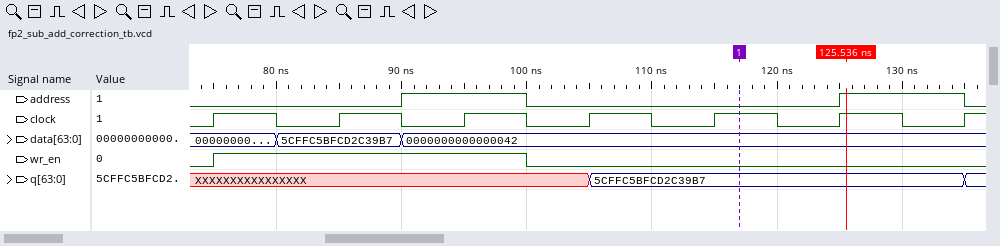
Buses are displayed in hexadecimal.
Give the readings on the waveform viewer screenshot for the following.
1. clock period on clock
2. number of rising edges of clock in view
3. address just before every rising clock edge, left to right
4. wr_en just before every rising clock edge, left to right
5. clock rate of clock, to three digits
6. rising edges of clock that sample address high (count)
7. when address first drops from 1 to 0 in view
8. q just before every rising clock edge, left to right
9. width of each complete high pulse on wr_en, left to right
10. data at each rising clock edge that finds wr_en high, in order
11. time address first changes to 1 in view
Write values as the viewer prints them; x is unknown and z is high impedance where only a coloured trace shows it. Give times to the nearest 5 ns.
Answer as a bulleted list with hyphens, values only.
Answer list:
- 10 ns
- 7
- 0 0 1 0 0 0 1
- 0 1 1 0 0 0 0
- 100 MHz
- 2
- 100 ns
- XXXXXXXXXXXXXXXX, XXXXXXXXXXXXXXXX, XXXXXXXXXXXXXXXX, XXXXXXXXXXXXXXXX, 5CFFC5BFCD2C39B7, 5CFFC5BFCD2C39B7, 5CFFC5BFCD2C39B7
- 25 ns
- 5CFFC5BFCD2C39B7, 0000000000000042
- 90 ns
